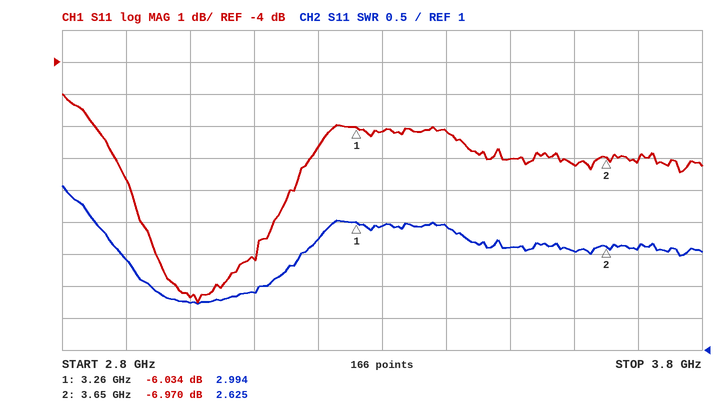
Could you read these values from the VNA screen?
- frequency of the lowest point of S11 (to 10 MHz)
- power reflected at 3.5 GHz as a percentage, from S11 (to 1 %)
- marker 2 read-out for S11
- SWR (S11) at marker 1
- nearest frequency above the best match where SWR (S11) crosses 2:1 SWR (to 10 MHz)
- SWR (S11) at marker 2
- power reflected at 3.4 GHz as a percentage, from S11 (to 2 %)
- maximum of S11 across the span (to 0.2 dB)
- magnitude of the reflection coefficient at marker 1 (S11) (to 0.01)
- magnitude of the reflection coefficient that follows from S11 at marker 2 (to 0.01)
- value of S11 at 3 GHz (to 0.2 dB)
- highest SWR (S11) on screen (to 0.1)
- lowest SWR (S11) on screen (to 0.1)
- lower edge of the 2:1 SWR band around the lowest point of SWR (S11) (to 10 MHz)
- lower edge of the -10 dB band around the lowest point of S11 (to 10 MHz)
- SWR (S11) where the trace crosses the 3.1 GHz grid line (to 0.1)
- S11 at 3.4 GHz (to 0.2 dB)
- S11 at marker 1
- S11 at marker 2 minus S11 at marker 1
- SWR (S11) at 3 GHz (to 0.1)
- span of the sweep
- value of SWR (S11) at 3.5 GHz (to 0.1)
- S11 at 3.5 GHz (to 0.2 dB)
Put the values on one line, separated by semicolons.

3.01 GHz; 20 %; -6.970 dB; 2.994; 3.11 GHz; 2.625; 24 %; -5.0 dB; 0.50; 0.45; -11.4 dB; 3.6; 1.7; 2.94 GHz; 2.95 GHz; 1.9; -6.2 dB; -6.034 dB; -0.936 dB; 1.7; 1 GHz; 2.6; -7.0 dB
